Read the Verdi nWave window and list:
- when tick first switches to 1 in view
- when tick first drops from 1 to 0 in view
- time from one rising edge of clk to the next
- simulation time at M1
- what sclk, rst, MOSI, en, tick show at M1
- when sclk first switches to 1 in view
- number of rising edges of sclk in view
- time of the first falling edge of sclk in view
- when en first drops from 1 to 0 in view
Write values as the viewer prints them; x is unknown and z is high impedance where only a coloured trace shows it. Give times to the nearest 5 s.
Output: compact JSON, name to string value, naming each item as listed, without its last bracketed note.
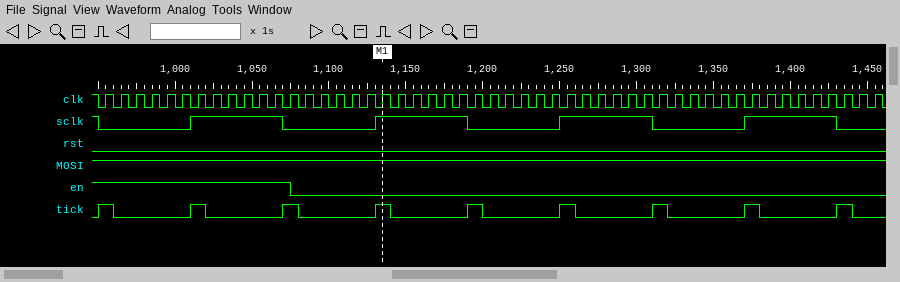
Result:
{"when tick first switches to 1 in view": "950 s", "when tick first drops from 1 to 0 in view": "960 s", "time from one rising edge of clk to the next": "10 s", "simulation time at M1": "1135 s", "what sclk, rst, MOSI, en, tick show at M1": "sclk=1, rst=0, MOSI=1, en=0, tick=1", "when sclk first switches to 1 in view": "1010 s", "number of rising edges of sclk in view": "4", "time of the first falling edge of sclk in view": "950 s", "when en first drops from 1 to 0 in view": "1075 s"}
